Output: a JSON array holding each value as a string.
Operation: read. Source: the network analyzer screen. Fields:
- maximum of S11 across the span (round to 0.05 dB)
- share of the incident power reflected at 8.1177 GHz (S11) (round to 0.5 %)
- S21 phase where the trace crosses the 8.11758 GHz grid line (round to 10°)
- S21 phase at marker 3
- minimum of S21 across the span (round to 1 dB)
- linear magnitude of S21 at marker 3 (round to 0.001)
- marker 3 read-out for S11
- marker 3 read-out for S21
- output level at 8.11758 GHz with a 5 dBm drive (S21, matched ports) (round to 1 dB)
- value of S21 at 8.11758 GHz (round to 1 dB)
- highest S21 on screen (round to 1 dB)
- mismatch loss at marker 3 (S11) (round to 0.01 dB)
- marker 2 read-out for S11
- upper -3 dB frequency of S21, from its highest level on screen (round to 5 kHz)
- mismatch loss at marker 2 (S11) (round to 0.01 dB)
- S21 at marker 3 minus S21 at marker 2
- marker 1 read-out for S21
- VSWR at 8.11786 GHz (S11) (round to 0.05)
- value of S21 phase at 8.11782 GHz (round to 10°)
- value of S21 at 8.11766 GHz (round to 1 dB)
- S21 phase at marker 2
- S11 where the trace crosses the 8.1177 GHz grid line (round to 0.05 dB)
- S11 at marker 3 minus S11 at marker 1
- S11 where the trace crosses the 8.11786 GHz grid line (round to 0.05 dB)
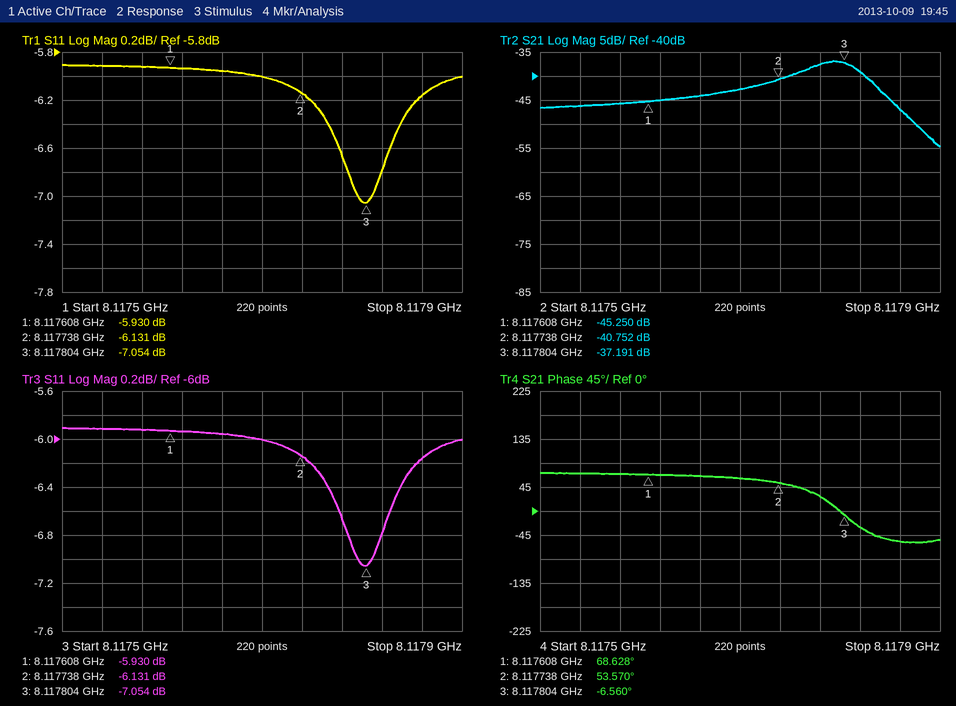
["-5.90 dB", "25.0 %", "70°", "-6.560°", "-55 dB", "0.014", "-7.054 dB", "-37.191 dB", "-41 dBm", "-46 dB", "-37 dB", "0.95 dB", "-6.131 dB", "8.117825 GHz", "1.21 dB", "3.561 dB", "-45.250 dB", "2.95", "-30°", "-44 dB", "53.570°", "-6.00 dB", "-1.124 dB", "-6.15 dB"]
